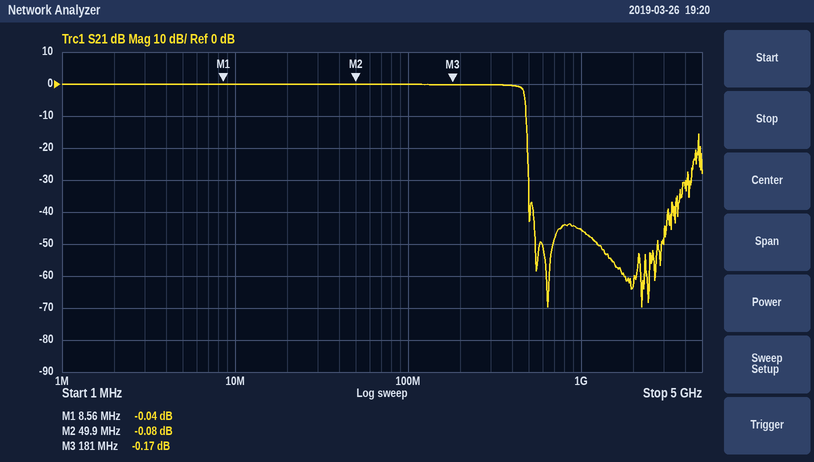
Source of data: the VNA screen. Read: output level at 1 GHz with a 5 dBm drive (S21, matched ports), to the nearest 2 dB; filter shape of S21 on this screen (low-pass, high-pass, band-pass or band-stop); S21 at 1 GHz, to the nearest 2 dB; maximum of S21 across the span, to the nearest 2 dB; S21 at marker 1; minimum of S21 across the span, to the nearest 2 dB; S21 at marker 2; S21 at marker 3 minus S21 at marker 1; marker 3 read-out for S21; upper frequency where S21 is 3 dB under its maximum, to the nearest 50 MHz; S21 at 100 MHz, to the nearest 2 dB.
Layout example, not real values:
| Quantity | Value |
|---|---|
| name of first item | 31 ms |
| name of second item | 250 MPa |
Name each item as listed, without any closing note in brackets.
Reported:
| Quantity | Value |
|---|---|
| output level at 1 GHz with a 5 dBm drive (S21, matched ports), to the nearest 2 dB | -40 dBm |
| filter shape of S21 on this screen | low-pass |
| S21 at 1 GHz, to the nearest 2 dB | -46 dB |
| maximum of S21 across the span, to the nearest 2 dB | 0 dB |
| S21 at marker 1 | -0.04 dB |
| minimum of S21 across the span, to the nearest 2 dB | -70 dB |
| S21 at marker 2 | -0.08 dB |
| S21 at marker 3 minus S21 at marker 1 | -0.13 dB |
| marker 3 read-out for S21 | -0.17 dB |
| upper frequency where S21 is 3 dB under its maximum, to the nearest 50 MHz | 450 MHz |
| S21 at 100 MHz, to the nearest 2 dB | 0 dB |
